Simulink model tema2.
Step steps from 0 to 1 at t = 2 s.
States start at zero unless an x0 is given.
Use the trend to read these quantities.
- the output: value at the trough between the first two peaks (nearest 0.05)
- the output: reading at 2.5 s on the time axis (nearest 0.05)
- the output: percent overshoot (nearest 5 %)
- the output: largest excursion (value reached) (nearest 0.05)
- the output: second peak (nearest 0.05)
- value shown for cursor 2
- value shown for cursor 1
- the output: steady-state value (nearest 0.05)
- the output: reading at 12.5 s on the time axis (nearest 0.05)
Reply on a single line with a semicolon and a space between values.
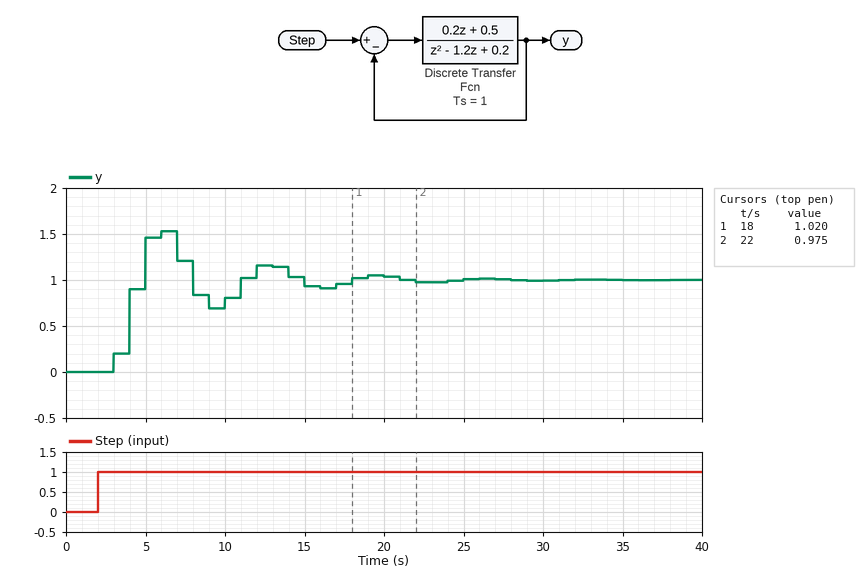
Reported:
0.70; 0.00; 55 %; 1.55; 1.15; 0.975; 1.020; 1.00; 1.15
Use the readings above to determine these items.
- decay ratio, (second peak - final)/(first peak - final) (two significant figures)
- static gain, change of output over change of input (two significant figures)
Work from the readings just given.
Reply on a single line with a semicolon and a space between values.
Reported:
0.27; 1.0
